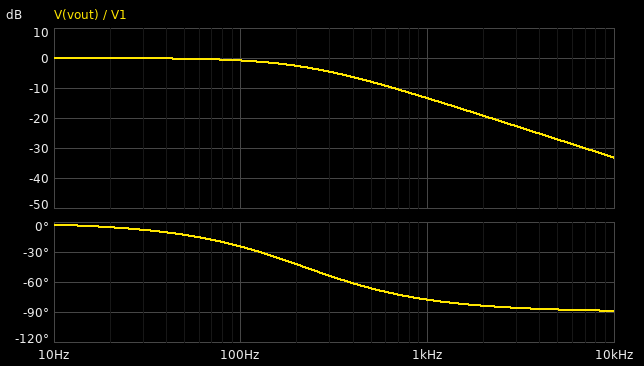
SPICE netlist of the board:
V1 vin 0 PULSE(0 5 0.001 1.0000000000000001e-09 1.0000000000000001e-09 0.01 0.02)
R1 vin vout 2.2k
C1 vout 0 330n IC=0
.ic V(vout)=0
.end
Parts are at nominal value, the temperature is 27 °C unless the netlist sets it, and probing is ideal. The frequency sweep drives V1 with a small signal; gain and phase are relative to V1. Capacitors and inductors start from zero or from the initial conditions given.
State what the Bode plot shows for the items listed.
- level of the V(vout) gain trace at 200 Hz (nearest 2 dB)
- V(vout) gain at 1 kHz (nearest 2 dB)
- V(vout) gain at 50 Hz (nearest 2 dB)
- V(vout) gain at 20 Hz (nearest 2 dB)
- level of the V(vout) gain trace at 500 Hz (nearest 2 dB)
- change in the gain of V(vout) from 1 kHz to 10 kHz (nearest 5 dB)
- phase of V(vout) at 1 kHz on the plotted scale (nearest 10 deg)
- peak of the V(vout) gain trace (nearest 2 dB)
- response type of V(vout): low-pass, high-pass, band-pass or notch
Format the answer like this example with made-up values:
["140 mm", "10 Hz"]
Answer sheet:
["-2 dB", "-14 dB", "0 dB", "0 dB", "-8 dB", "-20 dB", "-80 deg", "0 dB", "low-pass"]
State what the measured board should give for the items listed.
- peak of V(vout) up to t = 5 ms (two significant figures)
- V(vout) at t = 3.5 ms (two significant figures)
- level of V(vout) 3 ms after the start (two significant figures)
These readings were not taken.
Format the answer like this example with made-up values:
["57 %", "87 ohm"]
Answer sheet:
["5.0 V", "4.8 V", "4.7 V"]
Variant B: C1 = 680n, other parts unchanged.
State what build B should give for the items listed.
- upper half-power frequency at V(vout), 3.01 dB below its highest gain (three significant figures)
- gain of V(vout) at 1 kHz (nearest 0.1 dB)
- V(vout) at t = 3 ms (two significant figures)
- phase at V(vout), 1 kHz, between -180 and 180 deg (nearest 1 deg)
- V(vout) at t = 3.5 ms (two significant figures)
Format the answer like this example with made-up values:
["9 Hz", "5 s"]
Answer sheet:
["106 Hz", "-19.5 dB", "3.7 V", "-84 deg", "4.1 V"]
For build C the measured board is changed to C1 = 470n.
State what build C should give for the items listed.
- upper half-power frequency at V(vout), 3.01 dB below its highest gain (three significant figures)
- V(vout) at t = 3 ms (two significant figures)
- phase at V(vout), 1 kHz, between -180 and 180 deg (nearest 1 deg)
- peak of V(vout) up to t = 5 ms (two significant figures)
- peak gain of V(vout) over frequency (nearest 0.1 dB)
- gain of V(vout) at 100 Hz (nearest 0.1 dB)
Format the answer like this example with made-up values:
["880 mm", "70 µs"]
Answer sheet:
["154 Hz", "4.3 V", "-81 deg", "4.9 V", "0 dB", "-1.5 dB"]
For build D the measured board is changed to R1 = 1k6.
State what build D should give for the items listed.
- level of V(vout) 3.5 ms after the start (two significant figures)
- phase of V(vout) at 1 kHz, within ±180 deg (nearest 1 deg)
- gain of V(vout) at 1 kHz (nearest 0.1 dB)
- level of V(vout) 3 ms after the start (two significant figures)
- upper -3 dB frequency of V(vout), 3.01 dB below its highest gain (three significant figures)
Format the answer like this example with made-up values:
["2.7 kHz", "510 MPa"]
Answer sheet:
["5.0 V", "-73 deg", "-10.8 dB", "4.9 V", "301 Hz"]
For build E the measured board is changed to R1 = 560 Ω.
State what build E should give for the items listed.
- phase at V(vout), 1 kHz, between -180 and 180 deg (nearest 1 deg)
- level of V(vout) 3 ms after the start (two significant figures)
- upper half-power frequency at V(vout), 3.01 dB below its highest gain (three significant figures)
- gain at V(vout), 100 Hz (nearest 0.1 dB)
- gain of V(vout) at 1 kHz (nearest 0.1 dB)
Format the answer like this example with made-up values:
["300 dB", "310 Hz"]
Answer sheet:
["-49 deg", "5.0 V", "861 Hz", "-0.1 dB", "-3.7 dB"]
